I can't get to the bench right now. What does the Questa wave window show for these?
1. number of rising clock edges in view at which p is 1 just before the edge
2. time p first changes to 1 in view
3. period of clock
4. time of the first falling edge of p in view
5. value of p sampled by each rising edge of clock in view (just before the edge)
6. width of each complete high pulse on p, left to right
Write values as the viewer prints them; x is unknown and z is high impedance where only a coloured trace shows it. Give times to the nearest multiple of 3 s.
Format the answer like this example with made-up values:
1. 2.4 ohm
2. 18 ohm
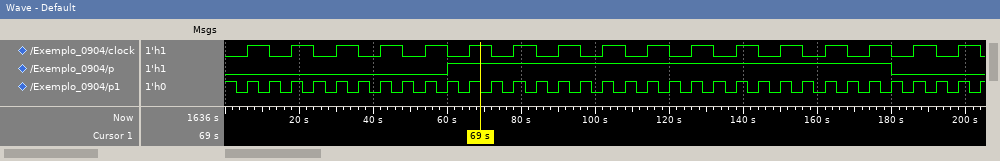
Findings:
1. 10
2. 60 s
3. 12 s
4. 180 s
5. 0 0 0 0 0 1 1 1 1 1 1 1 1 1 1 0 0
6. 120 s
